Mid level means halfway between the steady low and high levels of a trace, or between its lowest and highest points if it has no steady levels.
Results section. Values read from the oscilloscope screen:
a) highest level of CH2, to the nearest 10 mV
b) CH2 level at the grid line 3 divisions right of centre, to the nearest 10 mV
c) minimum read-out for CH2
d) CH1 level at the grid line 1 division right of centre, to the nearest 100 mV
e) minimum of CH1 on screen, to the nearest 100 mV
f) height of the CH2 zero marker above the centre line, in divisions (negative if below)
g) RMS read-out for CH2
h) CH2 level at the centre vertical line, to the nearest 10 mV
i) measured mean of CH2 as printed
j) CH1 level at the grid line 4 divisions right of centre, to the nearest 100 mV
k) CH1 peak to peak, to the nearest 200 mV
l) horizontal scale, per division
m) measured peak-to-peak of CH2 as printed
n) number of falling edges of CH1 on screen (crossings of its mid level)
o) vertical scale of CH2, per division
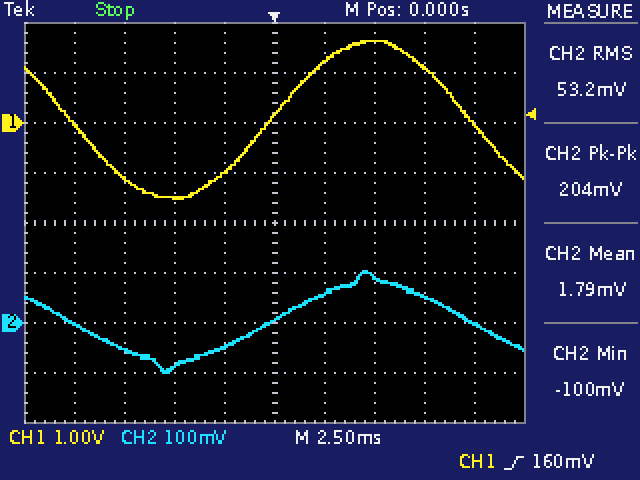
100 mV
50 mV
-100 mV
1.2 V
-1.5 V
-2.0 div
53.2 mV
10 mV
1.79 mV
0.0 V
3.2 V
2.5 ms
204 mV
2
100 mV
